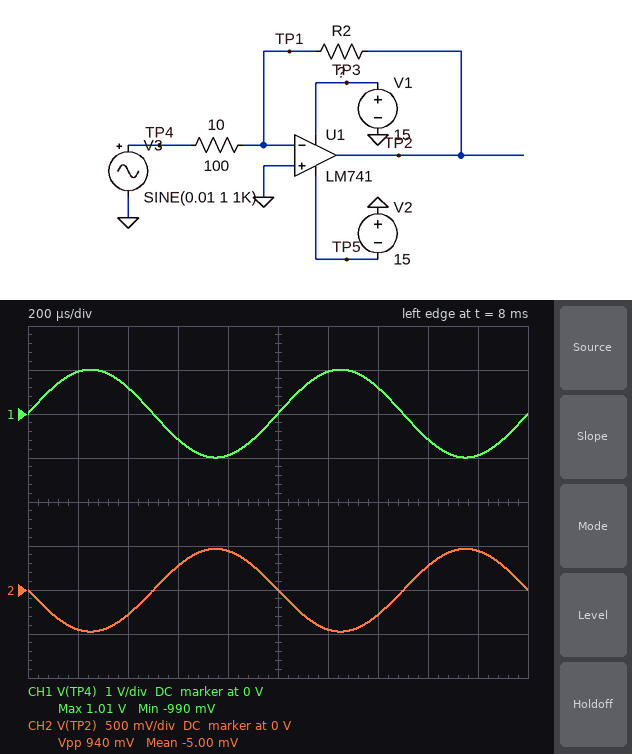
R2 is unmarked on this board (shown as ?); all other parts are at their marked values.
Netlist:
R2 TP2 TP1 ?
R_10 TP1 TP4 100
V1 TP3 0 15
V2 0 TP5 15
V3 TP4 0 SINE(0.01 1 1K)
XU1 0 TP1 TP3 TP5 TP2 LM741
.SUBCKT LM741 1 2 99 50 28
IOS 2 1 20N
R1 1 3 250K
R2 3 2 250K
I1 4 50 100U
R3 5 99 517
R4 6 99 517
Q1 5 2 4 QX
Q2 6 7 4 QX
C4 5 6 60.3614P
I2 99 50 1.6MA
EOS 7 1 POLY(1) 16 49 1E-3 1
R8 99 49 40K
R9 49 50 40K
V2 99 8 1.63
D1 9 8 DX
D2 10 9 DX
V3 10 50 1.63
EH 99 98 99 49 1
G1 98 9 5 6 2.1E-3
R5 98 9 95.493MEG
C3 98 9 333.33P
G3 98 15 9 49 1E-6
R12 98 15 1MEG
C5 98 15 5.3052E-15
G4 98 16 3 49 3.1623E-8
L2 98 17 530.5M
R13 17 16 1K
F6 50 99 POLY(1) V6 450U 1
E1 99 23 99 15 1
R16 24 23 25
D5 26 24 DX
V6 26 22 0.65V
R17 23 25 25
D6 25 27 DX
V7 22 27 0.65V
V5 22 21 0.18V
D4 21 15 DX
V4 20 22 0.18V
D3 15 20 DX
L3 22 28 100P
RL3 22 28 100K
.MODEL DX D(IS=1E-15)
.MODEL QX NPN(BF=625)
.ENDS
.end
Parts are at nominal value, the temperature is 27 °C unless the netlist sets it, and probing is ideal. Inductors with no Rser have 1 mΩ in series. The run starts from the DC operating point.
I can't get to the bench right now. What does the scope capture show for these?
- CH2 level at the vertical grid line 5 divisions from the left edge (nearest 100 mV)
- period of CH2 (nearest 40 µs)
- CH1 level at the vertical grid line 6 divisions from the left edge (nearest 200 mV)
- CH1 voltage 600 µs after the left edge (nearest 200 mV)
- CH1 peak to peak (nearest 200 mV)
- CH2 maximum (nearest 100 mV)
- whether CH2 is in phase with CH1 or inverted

0 V
1.00 ms
1.0 V
-600 mV
2.0 V
500 mV
inverted
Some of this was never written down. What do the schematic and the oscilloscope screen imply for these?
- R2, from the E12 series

47 Ω
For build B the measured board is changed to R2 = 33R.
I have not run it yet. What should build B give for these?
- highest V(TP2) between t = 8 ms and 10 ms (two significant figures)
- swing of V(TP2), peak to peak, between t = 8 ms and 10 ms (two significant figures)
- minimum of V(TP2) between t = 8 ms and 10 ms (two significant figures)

330 mV
660 mV
-330 mV
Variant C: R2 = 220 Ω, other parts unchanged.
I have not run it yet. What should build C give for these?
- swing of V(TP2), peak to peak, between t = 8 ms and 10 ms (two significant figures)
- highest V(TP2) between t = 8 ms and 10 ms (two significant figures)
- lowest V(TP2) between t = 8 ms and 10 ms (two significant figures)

4.4 V
2.2 V
-2.2 V
